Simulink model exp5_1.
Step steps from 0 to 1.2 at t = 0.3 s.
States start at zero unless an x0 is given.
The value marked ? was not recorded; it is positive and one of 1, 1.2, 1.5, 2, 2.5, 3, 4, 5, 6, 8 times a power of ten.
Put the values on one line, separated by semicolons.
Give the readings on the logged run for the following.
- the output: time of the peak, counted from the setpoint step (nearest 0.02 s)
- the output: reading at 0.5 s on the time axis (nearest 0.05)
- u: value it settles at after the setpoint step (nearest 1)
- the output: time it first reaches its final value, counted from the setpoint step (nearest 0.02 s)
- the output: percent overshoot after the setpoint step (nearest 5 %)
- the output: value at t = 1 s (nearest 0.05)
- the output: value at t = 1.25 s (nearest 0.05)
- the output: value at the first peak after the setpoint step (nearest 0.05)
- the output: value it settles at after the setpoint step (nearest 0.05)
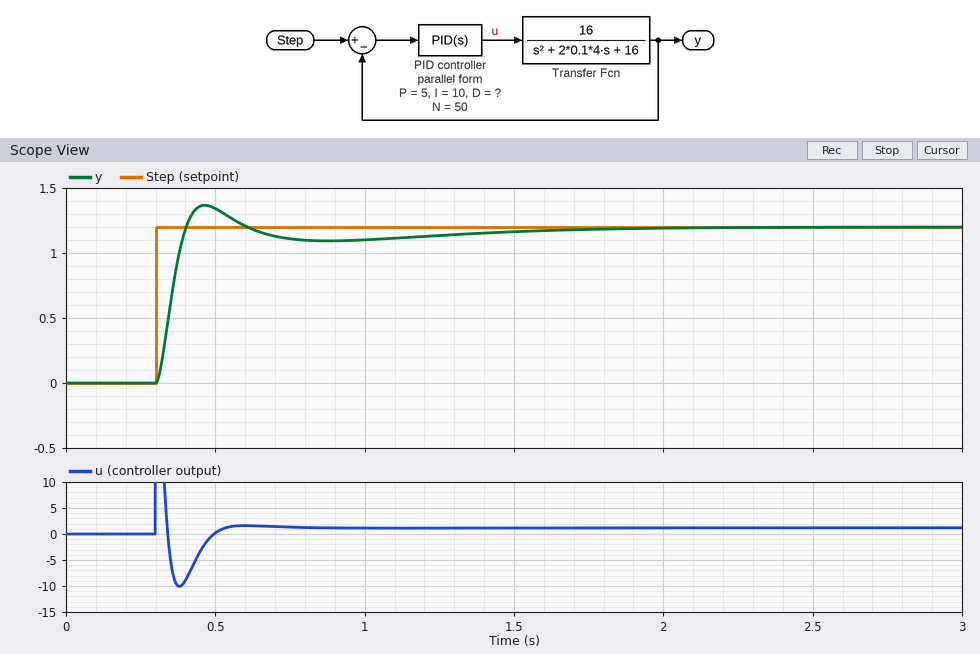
0.16 s; 1.35; 1; 0.10 s; 15 %; 1.10; 1.15; 1.35; 1.20
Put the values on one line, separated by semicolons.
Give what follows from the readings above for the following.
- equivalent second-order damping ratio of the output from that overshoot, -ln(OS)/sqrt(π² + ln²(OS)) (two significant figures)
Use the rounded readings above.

0.52
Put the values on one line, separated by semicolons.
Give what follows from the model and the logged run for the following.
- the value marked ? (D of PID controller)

1
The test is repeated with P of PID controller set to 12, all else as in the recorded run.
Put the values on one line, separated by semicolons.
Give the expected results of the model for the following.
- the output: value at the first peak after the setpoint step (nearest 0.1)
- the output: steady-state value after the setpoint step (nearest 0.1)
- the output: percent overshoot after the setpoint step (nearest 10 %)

1.6; 1.2; 30 %
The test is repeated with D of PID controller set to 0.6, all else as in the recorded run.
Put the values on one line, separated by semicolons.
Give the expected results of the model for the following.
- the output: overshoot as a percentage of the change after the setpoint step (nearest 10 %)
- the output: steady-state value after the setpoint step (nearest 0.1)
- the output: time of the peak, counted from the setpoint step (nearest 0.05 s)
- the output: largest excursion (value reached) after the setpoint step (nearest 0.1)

20 %; 1.2; 0.20 s; 1.5
